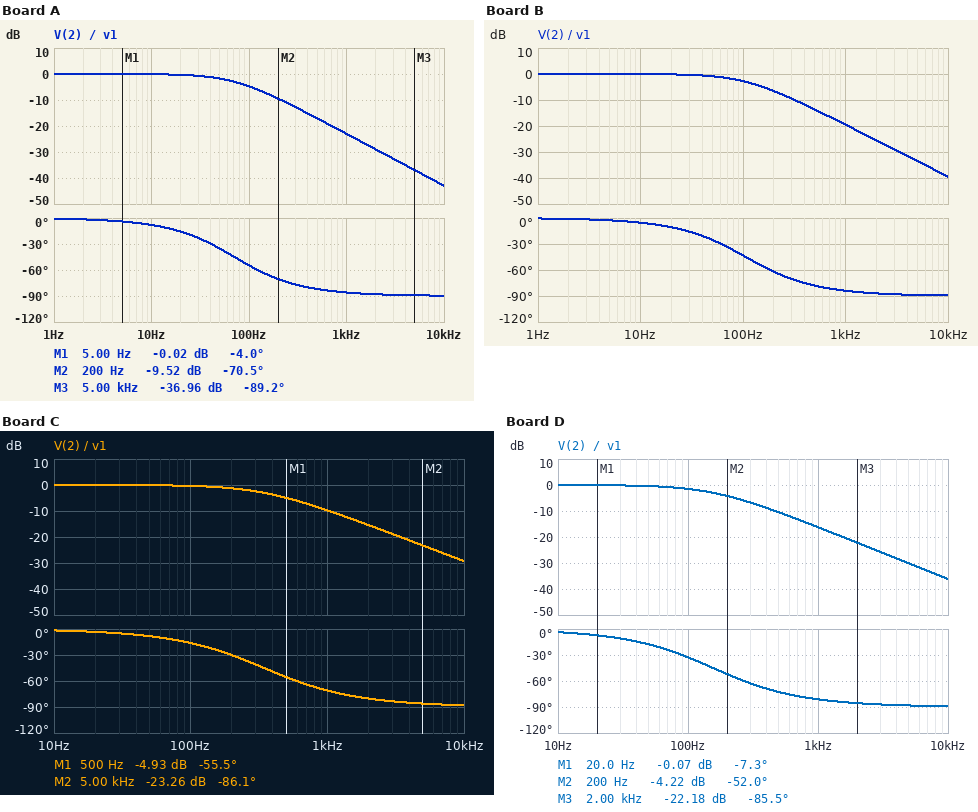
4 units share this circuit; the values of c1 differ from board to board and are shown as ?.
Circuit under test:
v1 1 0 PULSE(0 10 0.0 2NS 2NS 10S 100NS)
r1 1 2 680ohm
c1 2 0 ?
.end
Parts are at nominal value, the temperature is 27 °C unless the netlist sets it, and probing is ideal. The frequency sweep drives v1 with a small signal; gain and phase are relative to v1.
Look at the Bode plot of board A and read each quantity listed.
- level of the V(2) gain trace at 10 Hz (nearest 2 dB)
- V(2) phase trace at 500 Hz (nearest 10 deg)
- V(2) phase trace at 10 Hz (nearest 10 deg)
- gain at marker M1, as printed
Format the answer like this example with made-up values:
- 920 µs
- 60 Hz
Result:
- 0 dB
- -80 deg
- -10 deg
- -0.02 dB
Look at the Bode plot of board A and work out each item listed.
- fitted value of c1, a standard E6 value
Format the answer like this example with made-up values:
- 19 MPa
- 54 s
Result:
- 3.3 µF
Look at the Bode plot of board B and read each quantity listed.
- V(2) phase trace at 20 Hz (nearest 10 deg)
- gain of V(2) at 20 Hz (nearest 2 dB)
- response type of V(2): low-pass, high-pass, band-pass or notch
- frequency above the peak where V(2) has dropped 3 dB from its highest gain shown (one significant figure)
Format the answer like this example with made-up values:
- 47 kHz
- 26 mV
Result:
- -10 deg
- 0 dB
- low-pass
- 100 Hz
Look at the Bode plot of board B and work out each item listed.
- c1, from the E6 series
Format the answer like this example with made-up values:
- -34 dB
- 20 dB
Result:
- 2.2 µF
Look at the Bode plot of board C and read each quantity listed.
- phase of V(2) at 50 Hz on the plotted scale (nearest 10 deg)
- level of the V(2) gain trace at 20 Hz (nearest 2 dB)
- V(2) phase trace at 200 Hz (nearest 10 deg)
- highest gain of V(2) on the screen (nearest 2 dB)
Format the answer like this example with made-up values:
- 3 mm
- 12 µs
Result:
- -10 deg
- 0 dB
- -30 deg
- 0 dB
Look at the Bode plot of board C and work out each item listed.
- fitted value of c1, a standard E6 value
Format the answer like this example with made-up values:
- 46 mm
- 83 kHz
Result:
- 680 nF
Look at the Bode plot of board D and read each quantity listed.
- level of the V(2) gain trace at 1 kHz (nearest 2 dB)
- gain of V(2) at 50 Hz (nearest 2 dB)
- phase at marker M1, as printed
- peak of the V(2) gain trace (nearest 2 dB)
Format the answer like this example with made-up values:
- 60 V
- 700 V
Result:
- -16 dB
- 0 dB
- -7.3 deg
- 0 dB
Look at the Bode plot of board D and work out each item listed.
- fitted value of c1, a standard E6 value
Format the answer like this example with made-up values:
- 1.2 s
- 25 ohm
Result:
- 1.5 µF
